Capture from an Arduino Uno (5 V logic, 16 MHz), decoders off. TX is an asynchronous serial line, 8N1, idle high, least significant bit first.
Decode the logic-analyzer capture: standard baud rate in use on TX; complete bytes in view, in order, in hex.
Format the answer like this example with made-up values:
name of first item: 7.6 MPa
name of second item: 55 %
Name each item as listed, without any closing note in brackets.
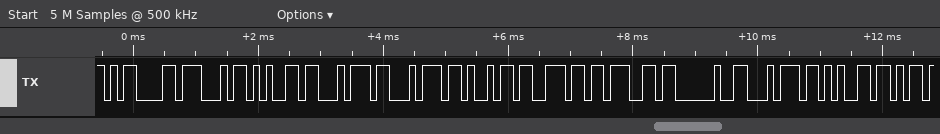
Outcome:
standard baud rate in use on TX: 9600 baud
complete bytes in view, in order, in hex: 0x0D 0x47 0x65 0x74 0x74 0x69 0x6E 0x67 0x20 0x74 0x65
